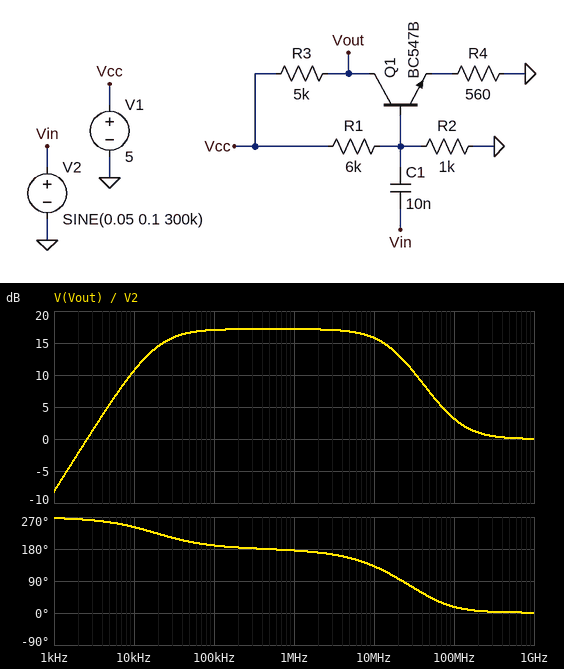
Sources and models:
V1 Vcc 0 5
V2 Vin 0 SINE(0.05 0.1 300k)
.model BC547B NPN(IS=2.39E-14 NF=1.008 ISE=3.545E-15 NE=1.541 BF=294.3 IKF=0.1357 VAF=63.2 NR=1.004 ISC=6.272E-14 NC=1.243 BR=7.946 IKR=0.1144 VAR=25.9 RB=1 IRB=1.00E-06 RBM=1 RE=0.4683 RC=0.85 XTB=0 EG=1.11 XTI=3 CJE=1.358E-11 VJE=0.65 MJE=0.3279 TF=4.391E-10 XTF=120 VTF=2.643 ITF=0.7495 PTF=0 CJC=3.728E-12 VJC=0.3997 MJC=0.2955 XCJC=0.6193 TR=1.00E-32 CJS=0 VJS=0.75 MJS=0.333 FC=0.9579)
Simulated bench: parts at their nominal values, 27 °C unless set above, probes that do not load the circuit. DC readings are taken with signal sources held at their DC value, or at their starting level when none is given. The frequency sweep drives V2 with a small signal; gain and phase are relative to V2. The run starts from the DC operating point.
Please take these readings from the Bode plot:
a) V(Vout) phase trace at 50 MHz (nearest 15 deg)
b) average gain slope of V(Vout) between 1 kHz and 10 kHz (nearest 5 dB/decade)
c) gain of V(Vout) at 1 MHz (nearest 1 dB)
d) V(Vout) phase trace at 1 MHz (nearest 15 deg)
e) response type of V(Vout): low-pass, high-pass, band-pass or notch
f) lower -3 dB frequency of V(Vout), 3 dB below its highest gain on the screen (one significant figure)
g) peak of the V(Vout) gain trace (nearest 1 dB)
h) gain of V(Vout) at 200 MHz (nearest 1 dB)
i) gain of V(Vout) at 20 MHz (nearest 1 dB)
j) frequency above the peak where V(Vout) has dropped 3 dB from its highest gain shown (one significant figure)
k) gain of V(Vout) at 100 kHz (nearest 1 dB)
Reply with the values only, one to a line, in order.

45 deg
20 dB/decade
17 dB
180 deg
band-pass
20 kHz
17 dB
1 dB
13 dB
20 MHz
17 dB
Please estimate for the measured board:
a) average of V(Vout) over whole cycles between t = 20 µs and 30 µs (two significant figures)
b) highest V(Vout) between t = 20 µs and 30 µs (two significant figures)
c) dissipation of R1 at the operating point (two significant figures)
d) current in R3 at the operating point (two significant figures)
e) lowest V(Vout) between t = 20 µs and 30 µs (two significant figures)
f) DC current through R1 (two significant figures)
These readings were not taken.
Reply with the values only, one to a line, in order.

3.9 V
4.6 V
3.1 mW
210 µA
3.2 V
710 µA
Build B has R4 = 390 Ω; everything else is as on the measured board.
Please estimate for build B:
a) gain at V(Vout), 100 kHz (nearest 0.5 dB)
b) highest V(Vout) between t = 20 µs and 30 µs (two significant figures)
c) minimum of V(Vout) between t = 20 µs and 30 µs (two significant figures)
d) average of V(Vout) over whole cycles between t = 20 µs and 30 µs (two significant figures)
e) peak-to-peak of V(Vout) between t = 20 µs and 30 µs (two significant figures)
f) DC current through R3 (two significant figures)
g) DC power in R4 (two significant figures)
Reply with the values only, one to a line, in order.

20.0 dB
4.5 V
2.5 V
3.6 V
2.0 V
280 µA
31 µW
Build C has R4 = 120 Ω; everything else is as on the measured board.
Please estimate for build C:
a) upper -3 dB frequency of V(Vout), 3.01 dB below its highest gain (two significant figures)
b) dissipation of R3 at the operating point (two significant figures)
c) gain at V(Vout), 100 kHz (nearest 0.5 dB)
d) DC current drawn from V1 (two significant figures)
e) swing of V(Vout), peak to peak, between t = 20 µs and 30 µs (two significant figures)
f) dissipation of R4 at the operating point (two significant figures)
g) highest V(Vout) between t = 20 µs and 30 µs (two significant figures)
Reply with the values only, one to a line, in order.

12 MHz
2.4 mW
29.5 dB
1.4 mA
4.3 V
58 µW
4.4 V
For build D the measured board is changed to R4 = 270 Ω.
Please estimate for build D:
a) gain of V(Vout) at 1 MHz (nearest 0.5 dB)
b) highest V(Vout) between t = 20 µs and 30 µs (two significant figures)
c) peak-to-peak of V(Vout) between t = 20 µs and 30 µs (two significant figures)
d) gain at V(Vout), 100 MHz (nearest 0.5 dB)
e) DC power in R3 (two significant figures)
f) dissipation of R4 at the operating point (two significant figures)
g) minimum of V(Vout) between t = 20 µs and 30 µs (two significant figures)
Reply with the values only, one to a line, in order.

23.0 dB
4.4 V
2.8 V
6.5 dB
700 µW
38 µW
1.6 V
